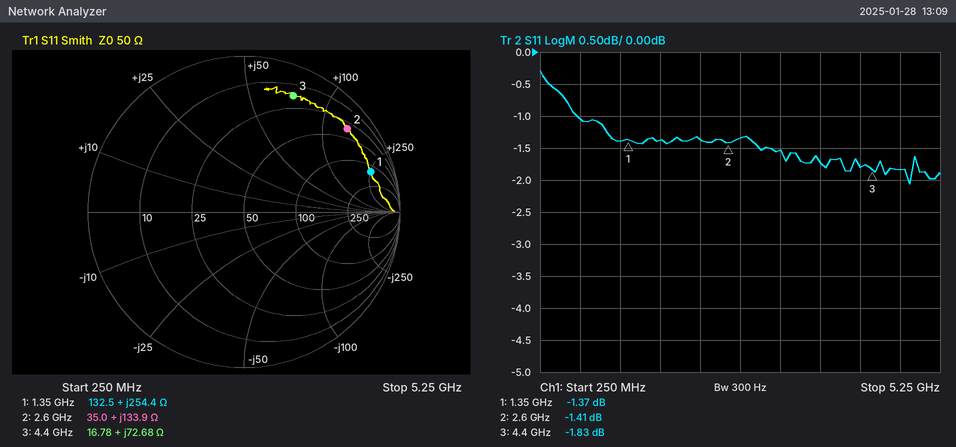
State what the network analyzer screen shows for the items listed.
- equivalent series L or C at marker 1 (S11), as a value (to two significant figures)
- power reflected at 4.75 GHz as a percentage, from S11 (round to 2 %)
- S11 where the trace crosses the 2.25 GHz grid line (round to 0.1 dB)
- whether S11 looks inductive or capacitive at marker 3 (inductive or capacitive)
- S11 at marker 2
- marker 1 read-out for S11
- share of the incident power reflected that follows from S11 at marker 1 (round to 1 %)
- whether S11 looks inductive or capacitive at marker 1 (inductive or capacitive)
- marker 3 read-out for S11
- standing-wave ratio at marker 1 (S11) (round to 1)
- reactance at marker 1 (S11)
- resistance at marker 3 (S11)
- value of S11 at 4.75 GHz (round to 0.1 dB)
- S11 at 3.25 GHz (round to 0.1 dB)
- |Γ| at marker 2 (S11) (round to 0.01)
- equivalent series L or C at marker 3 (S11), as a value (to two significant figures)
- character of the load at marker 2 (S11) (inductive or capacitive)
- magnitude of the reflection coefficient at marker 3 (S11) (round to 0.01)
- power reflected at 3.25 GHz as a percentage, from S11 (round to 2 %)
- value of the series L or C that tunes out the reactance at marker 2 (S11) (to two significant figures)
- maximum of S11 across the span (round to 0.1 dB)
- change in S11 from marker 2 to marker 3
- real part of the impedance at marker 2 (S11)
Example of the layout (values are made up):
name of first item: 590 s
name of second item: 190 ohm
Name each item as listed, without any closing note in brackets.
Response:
equivalent series L or C at marker 1 (S11), as a value: 30 nH
power reflected at 4.75 GHz as a percentage, from S11: 66 %
S11 where the trace crosses the 2.25 GHz grid line: -1.4 dB
whether S11 looks inductive or capacitive at marker 3: inductive
S11 at marker 2: -1.41 dB
marker 1 read-out for S11: -1.37 dB
share of the incident power reflected that follows from S11 at marker 1: 73 %
whether S11 looks inductive or capacitive at marker 1: inductive
marker 3 read-out for S11: -1.83 dB
standing-wave ratio at marker 1 (S11): 13
reactance at marker 1: +254.4 Ω
resistance at marker 3: 16.78 Ω
value of S11 at 4.75 GHz: -1.8 dB
S11 at 3.25 GHz: -1.5 dB
|Γ| at marker 2 (S11): 0.85
equivalent series L or C at marker 3 (S11), as a value: 2.6 nH
character of the load at marker 2 (S11): inductive
magnitude of the reflection coefficient at marker 3 (S11): 0.81
power reflected at 3.25 GHz as a percentage, from S11: 70 %
value of the series L or C that tunes out the reactance at marker 2 (S11): 460 fF
maximum of S11 across the span: -0.3 dB
change in S11 from marker 2 to marker 3: -0.42 dB
real part of the impedance at marker 2: 35.0 Ω
